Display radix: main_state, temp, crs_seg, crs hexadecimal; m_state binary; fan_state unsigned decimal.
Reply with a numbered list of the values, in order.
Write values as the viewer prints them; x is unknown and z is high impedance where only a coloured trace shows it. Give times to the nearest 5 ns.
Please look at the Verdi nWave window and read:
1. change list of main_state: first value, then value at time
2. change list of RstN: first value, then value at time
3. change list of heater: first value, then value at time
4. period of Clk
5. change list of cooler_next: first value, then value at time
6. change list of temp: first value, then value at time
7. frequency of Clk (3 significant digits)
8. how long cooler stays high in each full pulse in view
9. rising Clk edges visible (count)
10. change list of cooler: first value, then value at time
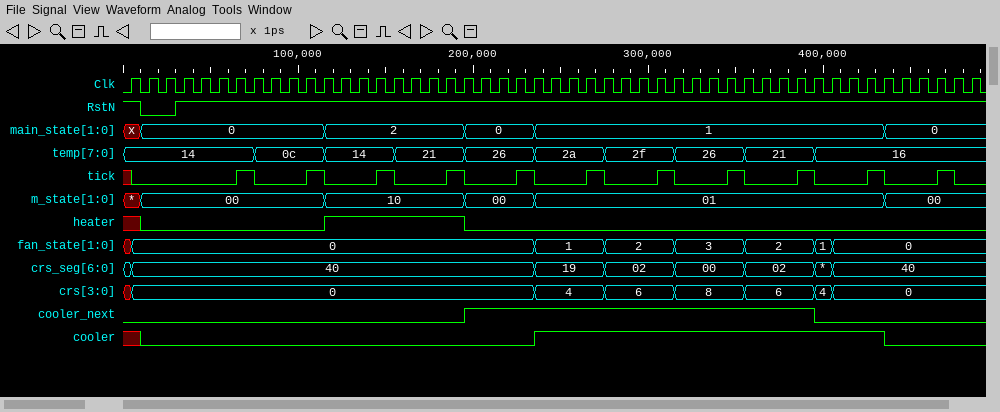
1. x, 0 at 10 ns, 2 at 115 ns, 0 at 195 ns, 1 at 235 ns, 0 at 435 ns
2. 1, 0 at 10 ns, 1 at 30 ns
3. x, 0 at 10 ns, 1 at 115 ns, 0 at 195 ns
4. 10 ns
5. 0, 1 at 195 ns, 0 at 395 ns
6. 14, 0c at 75 ns, 14 at 115 ns, 21 at 155 ns, 26 at 195 ns, 2a at 235 ns, 2f at 275 ns, 26 at 315 ns, 21 at 355 ns, 16 at 395 ns
7. 100 MHz
8. 200 ns
9. 49
10. x, 0 at 10 ns, 1 at 235 ns, 0 at 435 ns
